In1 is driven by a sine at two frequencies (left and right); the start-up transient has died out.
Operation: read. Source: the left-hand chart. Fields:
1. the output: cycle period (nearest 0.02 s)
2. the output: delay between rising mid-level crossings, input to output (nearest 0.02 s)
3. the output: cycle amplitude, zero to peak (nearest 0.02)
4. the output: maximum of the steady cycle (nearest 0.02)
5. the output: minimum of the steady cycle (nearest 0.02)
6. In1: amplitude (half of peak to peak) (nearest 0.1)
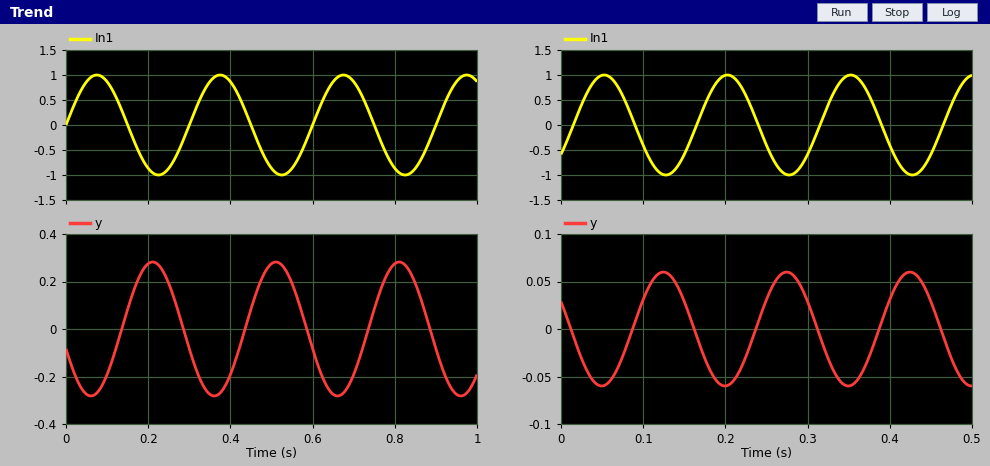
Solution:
0.30 s
0.14 s
0.28
0.28
-0.28
1.0
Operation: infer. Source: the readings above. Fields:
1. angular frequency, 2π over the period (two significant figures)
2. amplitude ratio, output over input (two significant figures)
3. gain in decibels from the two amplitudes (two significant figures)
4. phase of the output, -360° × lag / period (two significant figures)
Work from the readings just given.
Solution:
21 rad/s
0.28
-11 dB
-170°
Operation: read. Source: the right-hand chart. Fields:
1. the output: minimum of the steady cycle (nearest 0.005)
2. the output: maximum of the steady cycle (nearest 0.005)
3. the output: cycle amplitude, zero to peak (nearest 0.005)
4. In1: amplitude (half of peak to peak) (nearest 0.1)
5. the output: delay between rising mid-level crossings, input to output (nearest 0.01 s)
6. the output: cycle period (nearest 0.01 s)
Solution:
-0.060
0.060
0.060
1.0
0.07 s
0.15 s
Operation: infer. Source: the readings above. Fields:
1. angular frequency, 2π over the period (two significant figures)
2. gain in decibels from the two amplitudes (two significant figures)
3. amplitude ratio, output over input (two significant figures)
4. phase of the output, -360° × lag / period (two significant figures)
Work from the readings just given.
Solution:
42 rad/s
-24 dB
0.060
-170°
